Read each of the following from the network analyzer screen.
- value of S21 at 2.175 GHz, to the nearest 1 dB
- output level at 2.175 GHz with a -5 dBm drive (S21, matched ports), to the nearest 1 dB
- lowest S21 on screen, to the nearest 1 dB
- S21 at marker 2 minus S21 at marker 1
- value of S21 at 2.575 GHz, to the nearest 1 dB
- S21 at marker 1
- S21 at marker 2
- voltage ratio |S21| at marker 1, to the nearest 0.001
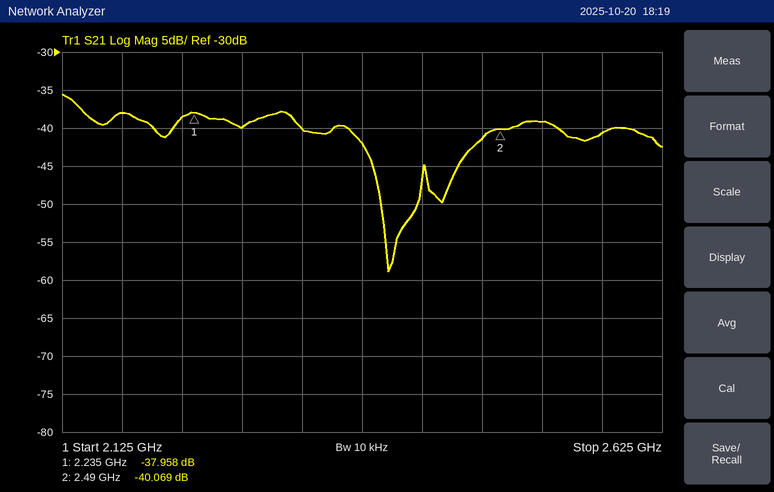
-38 dB
-43 dBm
-59 dB
-2.111 dB
-41 dB
-37.958 dB
-40.069 dB
0.013
